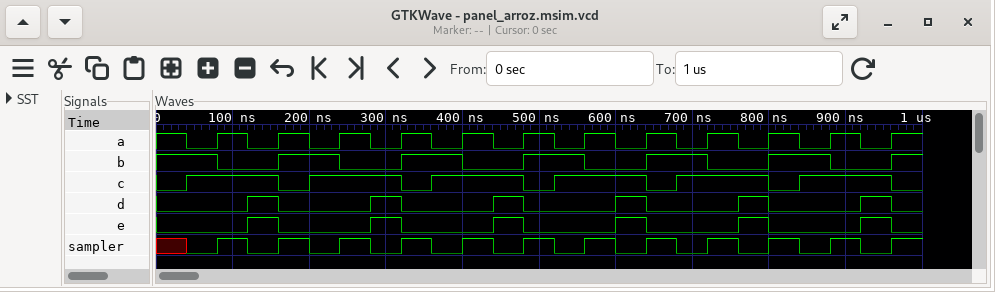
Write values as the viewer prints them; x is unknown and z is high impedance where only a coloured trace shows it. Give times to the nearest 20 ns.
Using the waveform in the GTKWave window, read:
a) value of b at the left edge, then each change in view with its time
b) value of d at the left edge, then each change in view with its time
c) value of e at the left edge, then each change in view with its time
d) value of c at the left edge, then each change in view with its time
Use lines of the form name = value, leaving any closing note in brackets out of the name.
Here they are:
value of b at the left edge, then each change in view with its time = 1, 0 at 80 ns, 1 at 160 ns, 0 at 240 ns, 1 at 320 ns, 0 at 400 ns, 1 at 480 ns, 0 at 560 ns, 1 at 640 ns, 0 at 720 ns, 1 at 800 ns, 0 at 880 ns, 1 at 960 ns
value of d at the left edge, then each change in view with its time = 0, 1 at 120 ns, 0 at 160 ns, 1 at 280 ns, 0 at 320 ns, 1 at 440 ns, 0 at 480 ns, 1 at 600 ns, 0 at 640 ns, 1 at 760 ns, 0 at 800 ns, 1 at 920 ns, 0 at 960 ns
value of e at the left edge, then each change in view with its time = 0, 1 at 120 ns, 0 at 160 ns, 1 at 280 ns, 0 at 320 ns, 1 at 440 ns, 0 at 480 ns, 1 at 600 ns, 0 at 640 ns, 1 at 760 ns, 0 at 800 ns, 1 at 920 ns, 0 at 960 ns
value of c at the left edge, then each change in view with its time = 0, 1 at 40 ns, 0 at 160 ns, 1 at 200 ns, 0 at 320 ns, 1 at 360 ns, 0 at 480 ns, 1 at 520 ns, 0 at 640 ns, 1 at 680 ns, 0 at 800 ns, 1 at 840 ns, 0 at 960 ns
